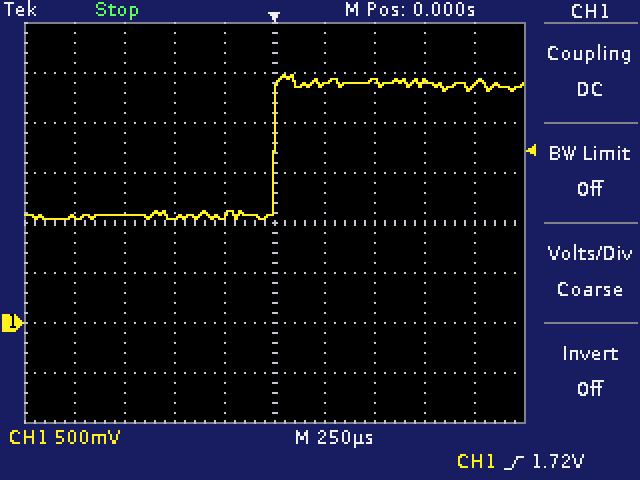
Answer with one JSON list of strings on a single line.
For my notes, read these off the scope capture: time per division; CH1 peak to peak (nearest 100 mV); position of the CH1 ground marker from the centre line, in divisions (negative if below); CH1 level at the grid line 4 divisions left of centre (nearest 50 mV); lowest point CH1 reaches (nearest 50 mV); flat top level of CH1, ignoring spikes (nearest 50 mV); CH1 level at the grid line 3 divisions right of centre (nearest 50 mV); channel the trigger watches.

["250 µs", "1.40 V", "-2.0 div", "1.05 V", "1.05 V", "2.40 V", "2.40 V", "CH1"]
